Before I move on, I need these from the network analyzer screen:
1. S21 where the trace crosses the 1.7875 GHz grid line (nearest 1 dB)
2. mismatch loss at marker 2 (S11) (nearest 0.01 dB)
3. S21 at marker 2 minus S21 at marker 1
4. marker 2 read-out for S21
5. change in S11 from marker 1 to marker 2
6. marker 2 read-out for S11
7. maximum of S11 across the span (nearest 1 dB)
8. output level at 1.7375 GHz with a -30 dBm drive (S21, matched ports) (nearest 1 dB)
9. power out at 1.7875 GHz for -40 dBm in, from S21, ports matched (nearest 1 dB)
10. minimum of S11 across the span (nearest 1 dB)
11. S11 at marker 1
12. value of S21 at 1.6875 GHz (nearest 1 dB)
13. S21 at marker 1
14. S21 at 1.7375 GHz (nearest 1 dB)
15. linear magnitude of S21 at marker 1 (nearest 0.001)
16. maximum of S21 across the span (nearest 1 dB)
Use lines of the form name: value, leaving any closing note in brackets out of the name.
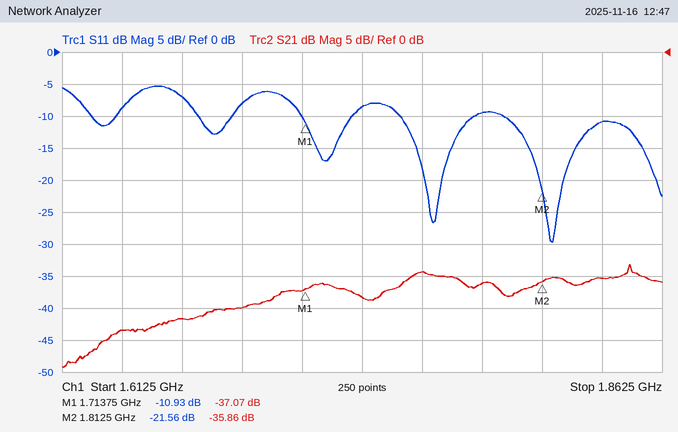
S21 where the trace crosses the 1.7875 GHz grid line: -36 dB
mismatch loss at marker 2 (S11): 0.03 dB
S21 at marker 2 minus S21 at marker 1: 1.21 dB
marker 2 read-out for S21: -35.86 dB
change in S11 from marker 1 to marker 2: -10.63 dB
marker 2 read-out for S11: -21.56 dB
maximum of S11 across the span: -5 dB
output level at 1.7375 GHz with a -30 dBm drive (S21, matched ports): -68 dBm
power out at 1.7875 GHz for -40 dBm in, from S21, ports matched: -76 dBm
minimum of S11 across the span: -30 dB
S11 at marker 1: -10.93 dB
value of S21 at 1.6875 GHz: -40 dB
S21 at marker 1: -37.07 dB
S21 at 1.7375 GHz: -38 dB
linear magnitude of S21 at marker 1: 0.014
maximum of S21 across the span: -33 dB
